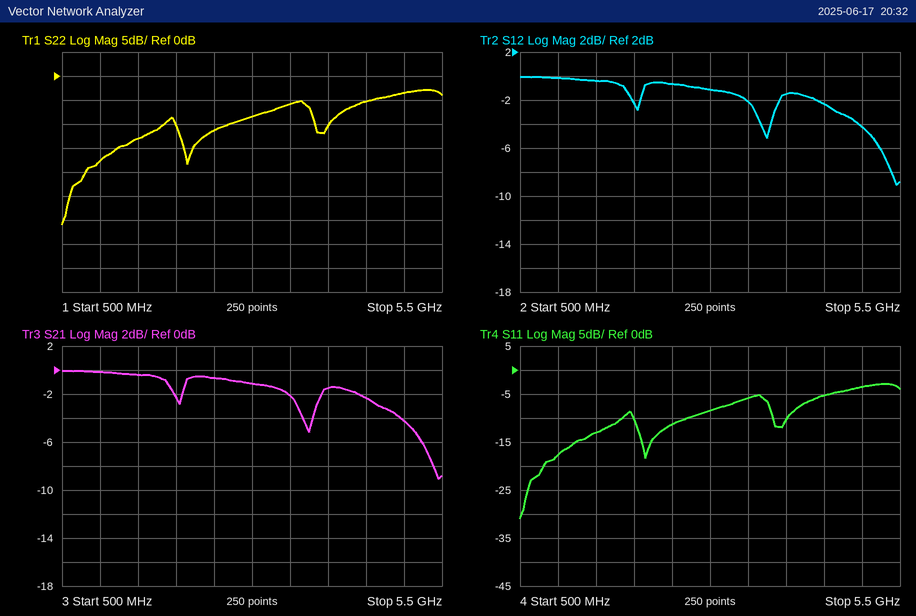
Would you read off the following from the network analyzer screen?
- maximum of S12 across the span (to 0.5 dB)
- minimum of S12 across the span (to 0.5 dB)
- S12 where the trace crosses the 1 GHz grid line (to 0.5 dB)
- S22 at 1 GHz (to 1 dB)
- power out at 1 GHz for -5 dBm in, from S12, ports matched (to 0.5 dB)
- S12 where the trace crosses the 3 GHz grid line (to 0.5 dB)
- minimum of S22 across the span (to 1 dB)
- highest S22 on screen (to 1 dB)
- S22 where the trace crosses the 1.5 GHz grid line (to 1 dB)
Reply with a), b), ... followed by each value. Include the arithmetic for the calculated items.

a) 0.0 dB
b) -9.0 dB
c) 0.0 dB
d) -18 dB
e) -5 dBm + (0.0 dB) = -5.0 dBm
f) -1.0 dB
g) -31 dB
h) -3 dB
i) -13 dB
